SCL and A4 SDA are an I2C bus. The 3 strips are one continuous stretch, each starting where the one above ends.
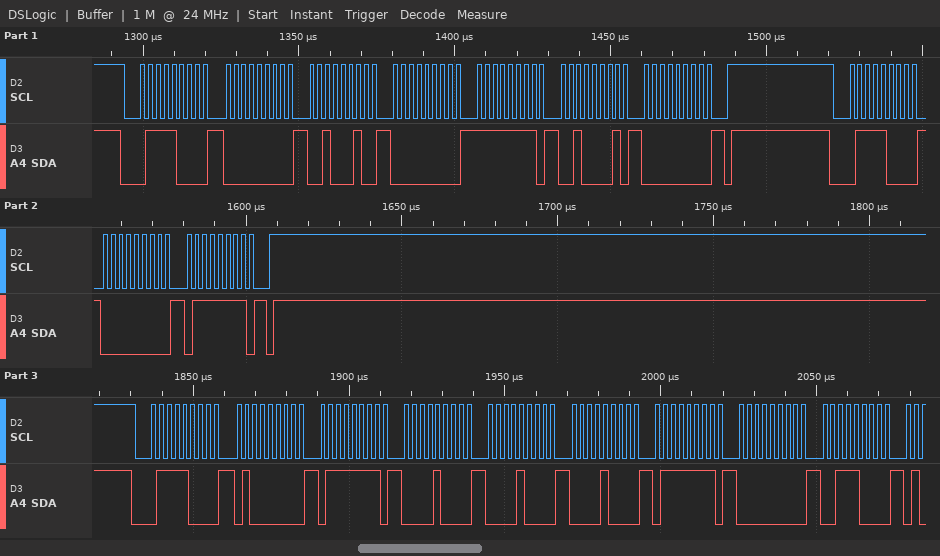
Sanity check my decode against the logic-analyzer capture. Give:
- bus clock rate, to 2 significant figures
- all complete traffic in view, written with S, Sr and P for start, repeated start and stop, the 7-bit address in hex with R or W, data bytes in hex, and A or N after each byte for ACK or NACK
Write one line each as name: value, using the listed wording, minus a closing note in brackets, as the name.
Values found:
bus clock rate, to 2 significant figures: 400 kHz
all complete traffic in view, written with S, Sr and P for start, repeated start and stop, the 7-bit address in hex with R or W, data bytes in hex, and A or N after each byte for ACK or NACK: S 3CW A 00 A 22 A 00 A FF A 21 A 00 A P S 3CW A 00 A 7F A P S 3CW A 40 A 7F A 08 A 08 A 08 A 7F A 00 A 38 A
